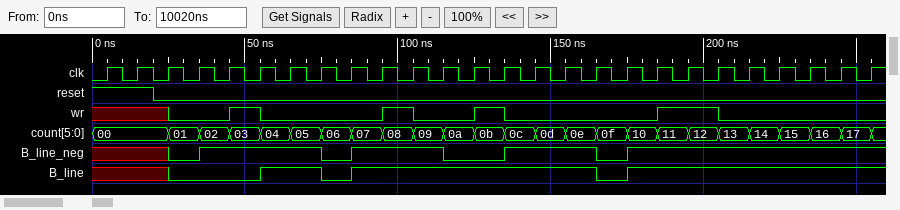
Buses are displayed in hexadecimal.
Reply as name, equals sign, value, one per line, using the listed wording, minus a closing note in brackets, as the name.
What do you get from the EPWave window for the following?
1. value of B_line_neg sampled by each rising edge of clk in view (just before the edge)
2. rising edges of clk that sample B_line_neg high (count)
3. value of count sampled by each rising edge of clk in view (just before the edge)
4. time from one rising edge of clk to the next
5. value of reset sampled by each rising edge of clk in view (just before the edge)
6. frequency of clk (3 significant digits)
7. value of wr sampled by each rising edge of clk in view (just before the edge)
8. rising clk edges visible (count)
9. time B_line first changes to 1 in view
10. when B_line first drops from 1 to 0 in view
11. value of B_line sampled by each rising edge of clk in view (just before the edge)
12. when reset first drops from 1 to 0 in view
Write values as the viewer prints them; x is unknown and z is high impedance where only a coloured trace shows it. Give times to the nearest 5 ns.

value of B_line_neg sampled by each rising edge of clk in view = x x x 0 1 1 1 1 0 1 1 1 0 0 1 1 1 0 1 1 1 1 1 1 1 1
rising edges of clk that sample B_line_neg high = 18
value of count sampled by each rising edge of clk in view = 00, 00, 00, 01, 02, 03, 04, 05, 06, 07, 08, 09, 0a, 0b, 0c, 0d, 0e, 0f, 10, 11, 12, 13, 14, 15, 16, 17
time from one rising edge of clk to the next = 10 ns
value of reset sampled by each rising edge of clk in view = 1 1 0 0 0 0 0 0 0 0 0 0 0 0 0 0 0 0 0 0 0 0 0 0 0 0
frequency of clk = 100 MHz
value of wr sampled by each rising edge of clk in view = x x x 0 0 1 0 0 0 0 1 0 0 1 0 0 0 0 0 1 1 0 0 0 0 0
rising clk edges visible = 26
time B_line first changes to 1 in view = 55 ns
when B_line first drops from 1 to 0 in view = 75 ns
value of B_line sampled by each rising edge of clk in view = x x x 0 0 0 1 1 0 1 1 1 1 1 1 1 1 0 1 1 1 1 1 1 1 1
when reset first drops from 1 to 0 in view = 20 ns
